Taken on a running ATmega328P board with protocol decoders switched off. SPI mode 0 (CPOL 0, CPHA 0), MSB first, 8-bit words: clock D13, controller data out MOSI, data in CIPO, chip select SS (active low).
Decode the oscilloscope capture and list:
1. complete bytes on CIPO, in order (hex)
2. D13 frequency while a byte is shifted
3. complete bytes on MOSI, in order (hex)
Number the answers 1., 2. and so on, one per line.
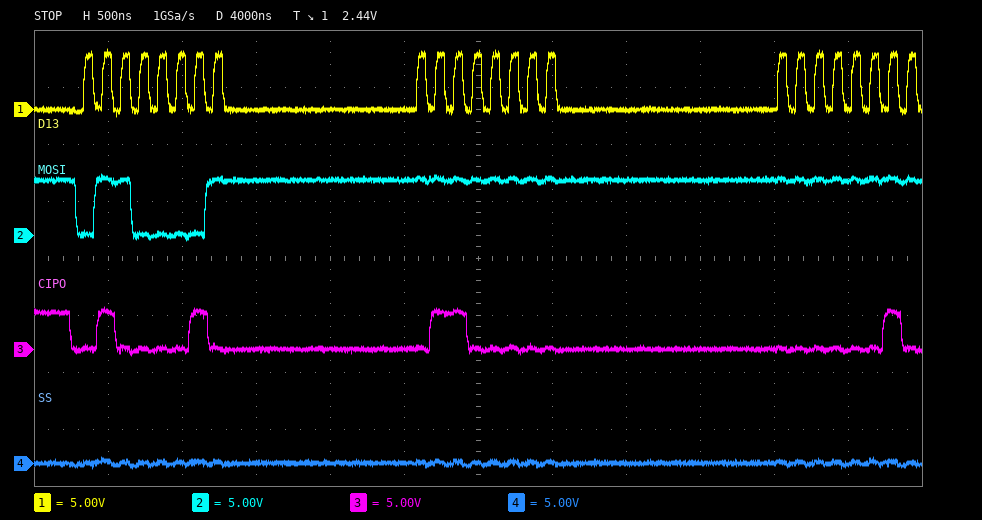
1. 42 60 02
2. 8 MHz
3. 61 FF FF
